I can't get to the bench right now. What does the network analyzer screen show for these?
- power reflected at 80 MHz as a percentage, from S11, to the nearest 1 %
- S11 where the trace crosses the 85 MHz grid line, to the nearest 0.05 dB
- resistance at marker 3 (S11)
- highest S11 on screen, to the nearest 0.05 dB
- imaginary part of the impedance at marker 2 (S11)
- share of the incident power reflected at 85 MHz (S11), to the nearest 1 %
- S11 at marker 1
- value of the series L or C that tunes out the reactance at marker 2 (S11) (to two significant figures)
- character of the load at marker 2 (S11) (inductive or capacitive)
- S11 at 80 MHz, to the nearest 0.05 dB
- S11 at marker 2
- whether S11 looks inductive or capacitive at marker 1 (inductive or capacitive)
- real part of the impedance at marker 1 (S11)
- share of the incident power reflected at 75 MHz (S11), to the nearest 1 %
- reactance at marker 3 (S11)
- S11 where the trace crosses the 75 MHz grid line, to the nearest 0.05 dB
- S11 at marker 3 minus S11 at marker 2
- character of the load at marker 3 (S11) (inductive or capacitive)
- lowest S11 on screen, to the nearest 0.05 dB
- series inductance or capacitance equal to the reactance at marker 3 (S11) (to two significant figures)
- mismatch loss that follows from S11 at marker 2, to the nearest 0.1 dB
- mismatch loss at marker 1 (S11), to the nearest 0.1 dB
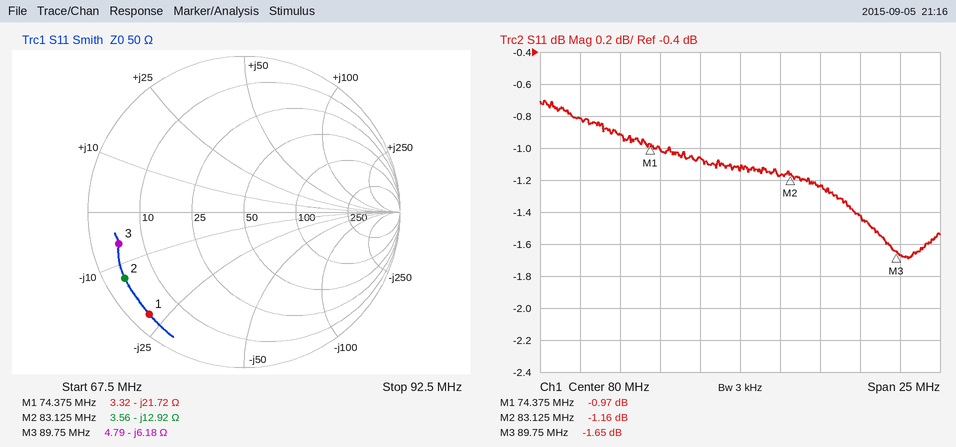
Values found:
77 %
-1.25 dB
4.79 Ω
-0.70 dB
-12.92 Ω
75 %
-0.97 dB
25 nH
capacitive
-1.15 dB
-1.16 dB
capacitive
3.32 Ω
79 %
-6.18 Ω
-1.00 dB
-0.49 dB
capacitive
-1.70 dB
290 pF
6.3 dB
7.0 dB
